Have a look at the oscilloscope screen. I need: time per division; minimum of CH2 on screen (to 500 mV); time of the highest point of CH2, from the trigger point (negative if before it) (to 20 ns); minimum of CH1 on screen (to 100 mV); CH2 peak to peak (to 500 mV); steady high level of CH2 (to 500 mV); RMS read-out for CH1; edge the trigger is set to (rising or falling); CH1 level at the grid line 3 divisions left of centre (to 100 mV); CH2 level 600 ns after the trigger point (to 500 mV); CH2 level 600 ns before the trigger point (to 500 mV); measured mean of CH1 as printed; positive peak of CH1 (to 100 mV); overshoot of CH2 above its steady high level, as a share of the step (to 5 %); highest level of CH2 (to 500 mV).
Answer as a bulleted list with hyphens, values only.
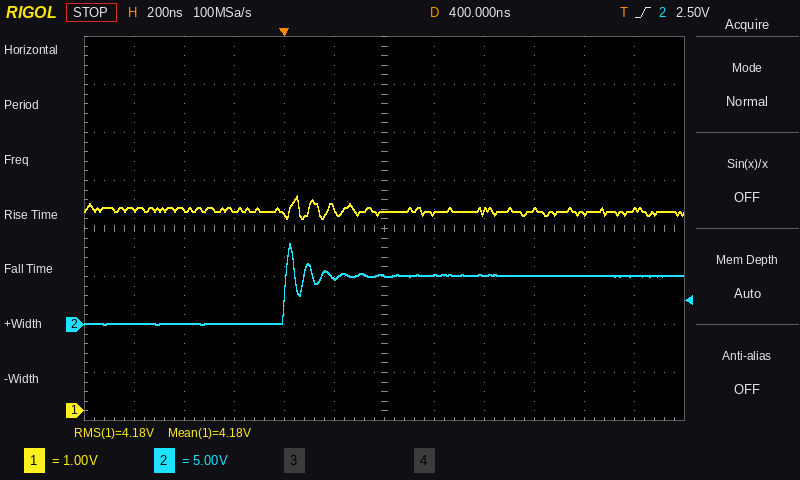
- 200 ns
- 0.0 V
- +20 ns
- 4.0 V
- 8.5 V
- 5.0 V
- 4.18 V
- rising
- 4.2 V
- 5.0 V
- 0.0 V
- 4.18 V
- 4.5 V
- 65 %
- 8.5 V
